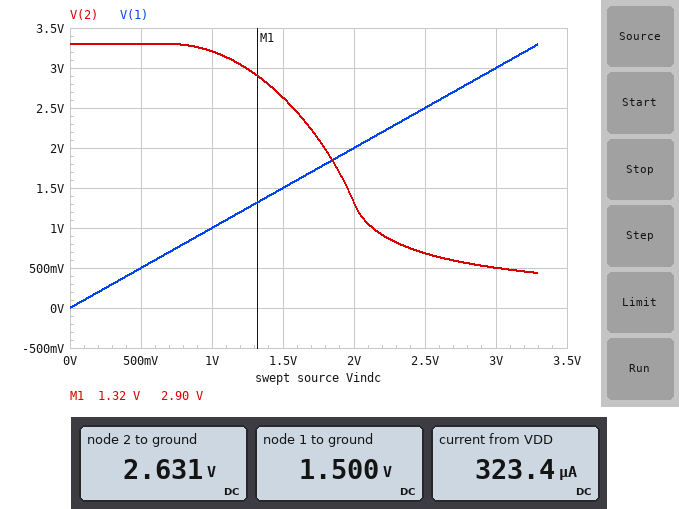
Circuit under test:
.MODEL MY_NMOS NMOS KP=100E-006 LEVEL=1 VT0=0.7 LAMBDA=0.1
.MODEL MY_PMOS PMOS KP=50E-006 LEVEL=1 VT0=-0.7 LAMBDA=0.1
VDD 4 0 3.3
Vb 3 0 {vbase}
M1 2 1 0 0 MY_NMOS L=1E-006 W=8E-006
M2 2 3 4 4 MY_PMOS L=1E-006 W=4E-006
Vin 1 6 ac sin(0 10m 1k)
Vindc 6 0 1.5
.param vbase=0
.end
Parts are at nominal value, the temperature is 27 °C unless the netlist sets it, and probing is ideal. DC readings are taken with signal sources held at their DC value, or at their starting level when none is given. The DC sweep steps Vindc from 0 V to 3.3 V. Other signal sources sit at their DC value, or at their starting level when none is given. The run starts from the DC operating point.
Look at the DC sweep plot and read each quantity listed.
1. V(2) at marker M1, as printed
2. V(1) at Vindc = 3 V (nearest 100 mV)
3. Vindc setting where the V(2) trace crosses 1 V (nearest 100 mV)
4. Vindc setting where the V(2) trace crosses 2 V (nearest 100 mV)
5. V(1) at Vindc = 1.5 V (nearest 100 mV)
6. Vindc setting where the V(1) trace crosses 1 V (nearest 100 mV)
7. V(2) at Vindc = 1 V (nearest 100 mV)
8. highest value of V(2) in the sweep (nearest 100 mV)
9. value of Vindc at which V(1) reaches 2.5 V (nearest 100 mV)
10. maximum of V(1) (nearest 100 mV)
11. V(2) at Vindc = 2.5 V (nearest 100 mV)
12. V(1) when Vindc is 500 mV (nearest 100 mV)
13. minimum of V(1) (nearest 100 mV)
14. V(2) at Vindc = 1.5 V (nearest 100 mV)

2.90 V
3.0 V
2.1 V
1.8 V
1.5 V
1.0 V
3.2 V
3.3 V
2.5 V
3.3 V
700 mV
500 mV
0 V
2.6 V
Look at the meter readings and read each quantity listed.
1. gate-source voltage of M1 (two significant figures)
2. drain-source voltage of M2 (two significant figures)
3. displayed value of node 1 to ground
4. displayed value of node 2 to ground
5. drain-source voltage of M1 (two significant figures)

1.5 V
-670 mV
1.500 V
2.631 V
2.6 V
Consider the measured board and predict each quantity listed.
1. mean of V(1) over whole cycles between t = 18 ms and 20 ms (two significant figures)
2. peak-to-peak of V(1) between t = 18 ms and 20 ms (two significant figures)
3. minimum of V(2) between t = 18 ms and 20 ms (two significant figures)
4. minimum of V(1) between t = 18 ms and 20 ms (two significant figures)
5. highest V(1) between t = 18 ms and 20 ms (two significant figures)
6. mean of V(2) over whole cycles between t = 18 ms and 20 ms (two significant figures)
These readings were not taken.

1.5 V
20 mV
2.6 V
1.5 V
1.5 V
2.6 V
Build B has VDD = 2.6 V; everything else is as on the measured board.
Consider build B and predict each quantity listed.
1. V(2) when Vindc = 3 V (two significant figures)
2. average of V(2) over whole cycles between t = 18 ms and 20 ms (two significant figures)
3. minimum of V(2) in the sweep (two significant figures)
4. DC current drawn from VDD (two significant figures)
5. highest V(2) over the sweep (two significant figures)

250 mV
1.6 V
220 mV
300 µA
2.6 V
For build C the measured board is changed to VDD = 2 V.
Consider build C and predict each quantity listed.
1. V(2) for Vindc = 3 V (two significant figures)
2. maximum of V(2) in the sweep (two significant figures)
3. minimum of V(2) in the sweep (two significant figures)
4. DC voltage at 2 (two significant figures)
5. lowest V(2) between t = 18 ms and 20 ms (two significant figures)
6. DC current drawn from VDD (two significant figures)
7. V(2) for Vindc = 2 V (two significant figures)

110 mV
2.0 V
98 mV
390 mV
380 mV
200 µA
200 mV
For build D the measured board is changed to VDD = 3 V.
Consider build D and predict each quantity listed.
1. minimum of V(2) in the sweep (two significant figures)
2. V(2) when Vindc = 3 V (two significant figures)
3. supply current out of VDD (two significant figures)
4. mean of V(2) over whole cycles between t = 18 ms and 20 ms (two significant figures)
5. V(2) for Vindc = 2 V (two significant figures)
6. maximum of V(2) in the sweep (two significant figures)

330 mV
380 mV
310 µA
2.2 V
840 mV
3.0 V
